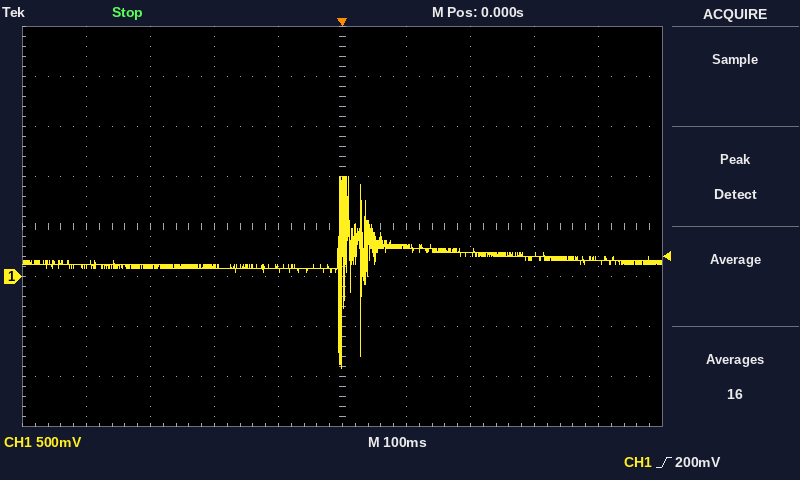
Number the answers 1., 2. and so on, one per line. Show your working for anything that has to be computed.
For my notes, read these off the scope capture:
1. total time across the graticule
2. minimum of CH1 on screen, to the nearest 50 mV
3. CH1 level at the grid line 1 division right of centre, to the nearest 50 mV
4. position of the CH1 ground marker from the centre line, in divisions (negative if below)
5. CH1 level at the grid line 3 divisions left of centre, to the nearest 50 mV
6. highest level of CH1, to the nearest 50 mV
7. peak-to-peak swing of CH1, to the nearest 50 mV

1. 1 s
2. -900 mV
3. 300 mV
4. -1.0 div
5. 100 mV
6. 1.00 V
7. 1.00 V − (-900 mV) = 1.90 V
